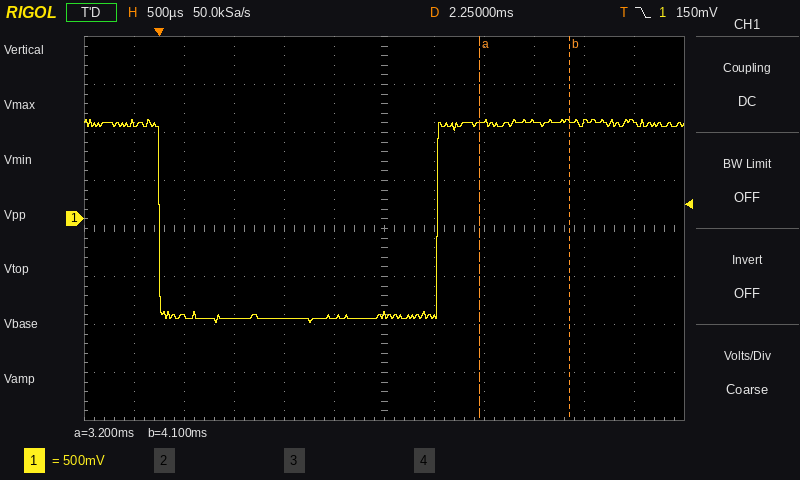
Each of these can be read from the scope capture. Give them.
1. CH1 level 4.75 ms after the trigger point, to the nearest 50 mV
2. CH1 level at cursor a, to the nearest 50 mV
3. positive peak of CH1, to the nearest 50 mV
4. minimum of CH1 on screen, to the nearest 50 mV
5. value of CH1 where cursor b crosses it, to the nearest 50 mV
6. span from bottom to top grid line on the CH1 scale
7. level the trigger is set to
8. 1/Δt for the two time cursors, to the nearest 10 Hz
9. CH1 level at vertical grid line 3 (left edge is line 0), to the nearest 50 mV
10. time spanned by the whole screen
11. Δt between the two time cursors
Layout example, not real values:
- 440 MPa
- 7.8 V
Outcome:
- 1.00 V
- 1.00 V
- 1.05 V
- -1.10 V
- 1.00 V
- 4 V
- 150 mV
- 1.11 kHz
- -1.05 V
- 6 ms
- 900 µs
